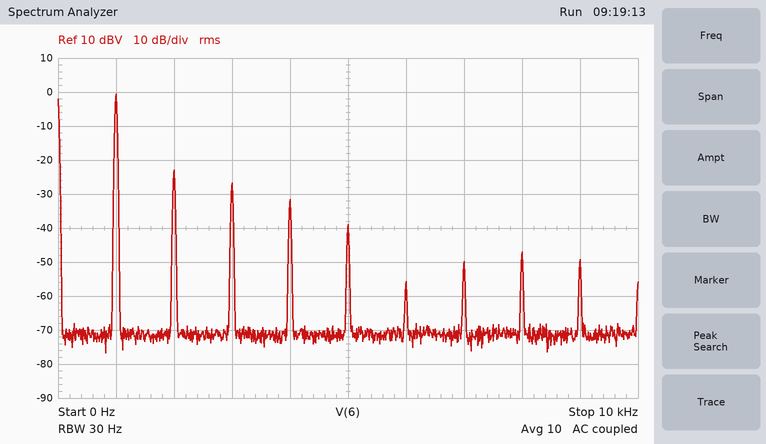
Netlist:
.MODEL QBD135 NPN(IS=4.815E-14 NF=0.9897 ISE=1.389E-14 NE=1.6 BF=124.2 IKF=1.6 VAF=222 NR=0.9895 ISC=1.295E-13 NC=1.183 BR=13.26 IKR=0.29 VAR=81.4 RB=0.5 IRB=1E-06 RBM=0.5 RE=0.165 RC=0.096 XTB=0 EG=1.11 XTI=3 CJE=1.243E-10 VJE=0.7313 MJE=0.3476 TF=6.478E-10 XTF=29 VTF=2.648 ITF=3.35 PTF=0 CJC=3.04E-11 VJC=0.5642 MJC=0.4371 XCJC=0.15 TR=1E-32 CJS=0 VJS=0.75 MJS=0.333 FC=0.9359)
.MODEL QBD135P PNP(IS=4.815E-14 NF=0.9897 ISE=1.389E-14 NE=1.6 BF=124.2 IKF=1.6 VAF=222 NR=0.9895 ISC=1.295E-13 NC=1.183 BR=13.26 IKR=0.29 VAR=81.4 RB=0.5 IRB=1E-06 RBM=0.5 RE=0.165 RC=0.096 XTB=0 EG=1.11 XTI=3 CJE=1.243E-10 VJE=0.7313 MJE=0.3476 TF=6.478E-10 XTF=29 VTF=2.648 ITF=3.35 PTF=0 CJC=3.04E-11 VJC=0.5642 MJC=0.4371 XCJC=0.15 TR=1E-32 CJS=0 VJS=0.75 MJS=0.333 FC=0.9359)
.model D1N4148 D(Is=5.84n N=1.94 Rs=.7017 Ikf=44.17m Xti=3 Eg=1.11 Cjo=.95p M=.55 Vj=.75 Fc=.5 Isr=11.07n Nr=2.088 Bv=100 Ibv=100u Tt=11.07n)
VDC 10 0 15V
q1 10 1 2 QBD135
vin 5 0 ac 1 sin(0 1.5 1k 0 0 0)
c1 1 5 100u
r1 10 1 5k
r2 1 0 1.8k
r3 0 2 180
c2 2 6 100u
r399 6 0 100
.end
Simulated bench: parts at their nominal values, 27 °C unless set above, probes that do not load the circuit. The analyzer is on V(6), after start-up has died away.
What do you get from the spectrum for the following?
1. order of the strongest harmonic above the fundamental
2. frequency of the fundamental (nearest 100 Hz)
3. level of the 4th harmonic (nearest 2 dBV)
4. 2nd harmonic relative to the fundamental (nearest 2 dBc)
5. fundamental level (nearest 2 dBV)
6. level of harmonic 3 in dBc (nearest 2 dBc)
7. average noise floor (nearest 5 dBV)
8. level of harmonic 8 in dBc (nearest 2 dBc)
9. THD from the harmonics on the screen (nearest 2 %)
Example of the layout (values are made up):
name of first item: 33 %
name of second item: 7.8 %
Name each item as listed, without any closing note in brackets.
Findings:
order of the strongest harmonic above the fundamental: 2
frequency of the fundamental: 1.0 kHz
level of the 4th harmonic: -32 dBV
2nd harmonic relative to the fundamental: -22 dBc
fundamental level: 0 dBV
level of harmonic 3 in dBc: -26 dBc
average noise floor: -70 dBV
level of harmonic 8 in dBc: -46 dBc
THD from the harmonics on the screen: 10 %
